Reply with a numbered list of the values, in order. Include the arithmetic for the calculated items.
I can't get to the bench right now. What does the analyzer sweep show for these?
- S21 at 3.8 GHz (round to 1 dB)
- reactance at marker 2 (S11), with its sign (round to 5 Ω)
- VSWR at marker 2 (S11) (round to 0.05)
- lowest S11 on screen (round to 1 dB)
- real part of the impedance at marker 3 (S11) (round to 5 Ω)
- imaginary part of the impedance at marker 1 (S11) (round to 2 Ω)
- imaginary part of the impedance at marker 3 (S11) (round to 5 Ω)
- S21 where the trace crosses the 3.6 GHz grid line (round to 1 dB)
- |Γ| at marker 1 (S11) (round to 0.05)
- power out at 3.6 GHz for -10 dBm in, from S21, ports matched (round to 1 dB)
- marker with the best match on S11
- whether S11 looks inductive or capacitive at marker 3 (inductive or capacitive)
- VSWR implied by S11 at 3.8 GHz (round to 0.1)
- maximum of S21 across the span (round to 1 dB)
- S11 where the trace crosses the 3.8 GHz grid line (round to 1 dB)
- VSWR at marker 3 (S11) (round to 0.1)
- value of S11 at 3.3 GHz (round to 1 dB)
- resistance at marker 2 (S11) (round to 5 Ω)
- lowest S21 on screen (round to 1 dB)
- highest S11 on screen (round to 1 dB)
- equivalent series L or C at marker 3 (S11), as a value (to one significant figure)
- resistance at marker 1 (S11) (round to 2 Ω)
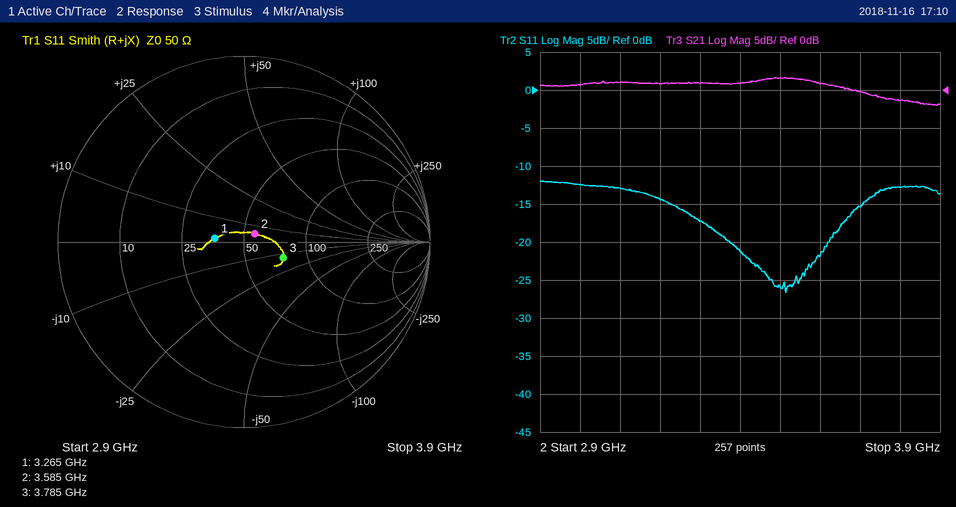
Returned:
1. -1 dB
2. +5 Ω
3. 1.15
4. -27 dB
5. 75 Ω
6. +2 Ω
7. -15 Ω
8. 1 dB
9. 0.15
10. -10 dBm + (1 dB) = -9 dBm
11. marker 2
12. capacitive
13. |Γ| = 10^(-13/20) = 0.2239; VSWR = (1 + 0.2239)/(1 − 0.2239) ≈ 1.6
14. 2 dB
15. -13 dB
16. 1.6
17. -17 dB
18. 55 Ω
19. -2 dB
20. -12 dB
21. C = 1/(2π × 3.785 GHz × 15 Ω) ≈ 3 pF
22. 36 Ω
